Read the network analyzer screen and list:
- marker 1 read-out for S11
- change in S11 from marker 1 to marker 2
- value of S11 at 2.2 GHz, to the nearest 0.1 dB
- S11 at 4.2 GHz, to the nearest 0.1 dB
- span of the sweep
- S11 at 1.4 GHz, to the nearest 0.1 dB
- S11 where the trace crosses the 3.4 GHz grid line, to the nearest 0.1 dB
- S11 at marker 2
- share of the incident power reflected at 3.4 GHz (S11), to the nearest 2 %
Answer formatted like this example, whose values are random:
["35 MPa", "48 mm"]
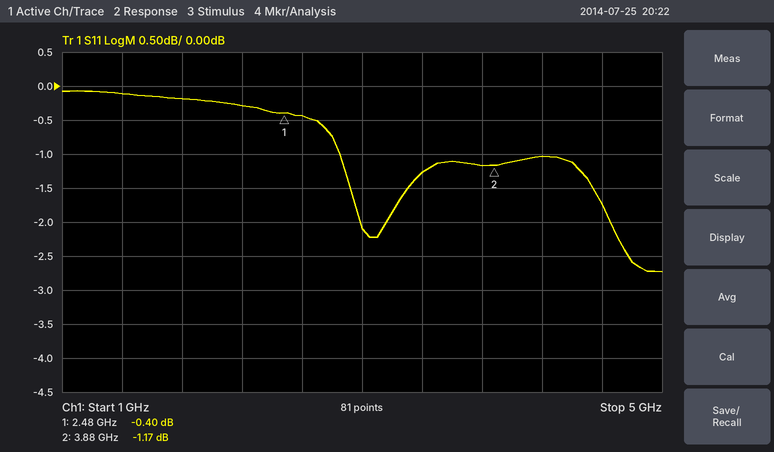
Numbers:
["-0.40 dB", "-0.77 dB", "-0.3 dB", "-1.0 dB", "4 GHz", "-0.1 dB", "-1.3 dB", "-1.17 dB", "74 %"]
